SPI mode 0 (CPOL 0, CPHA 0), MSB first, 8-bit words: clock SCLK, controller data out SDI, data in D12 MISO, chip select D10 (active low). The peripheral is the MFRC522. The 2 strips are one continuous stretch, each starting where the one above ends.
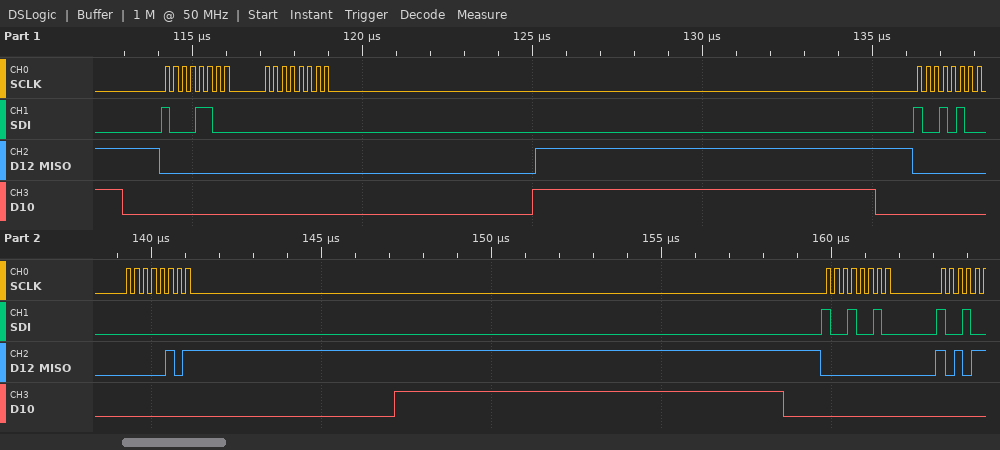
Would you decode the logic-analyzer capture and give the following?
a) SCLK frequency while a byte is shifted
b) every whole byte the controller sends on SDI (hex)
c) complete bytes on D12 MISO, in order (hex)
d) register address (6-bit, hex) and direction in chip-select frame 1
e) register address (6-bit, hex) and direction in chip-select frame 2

4 MHz
0x8C 0x00 0x94 0x00 0x92
0x00 0x00 0x00 0x05 0x00
0x06 read
0x0A read
